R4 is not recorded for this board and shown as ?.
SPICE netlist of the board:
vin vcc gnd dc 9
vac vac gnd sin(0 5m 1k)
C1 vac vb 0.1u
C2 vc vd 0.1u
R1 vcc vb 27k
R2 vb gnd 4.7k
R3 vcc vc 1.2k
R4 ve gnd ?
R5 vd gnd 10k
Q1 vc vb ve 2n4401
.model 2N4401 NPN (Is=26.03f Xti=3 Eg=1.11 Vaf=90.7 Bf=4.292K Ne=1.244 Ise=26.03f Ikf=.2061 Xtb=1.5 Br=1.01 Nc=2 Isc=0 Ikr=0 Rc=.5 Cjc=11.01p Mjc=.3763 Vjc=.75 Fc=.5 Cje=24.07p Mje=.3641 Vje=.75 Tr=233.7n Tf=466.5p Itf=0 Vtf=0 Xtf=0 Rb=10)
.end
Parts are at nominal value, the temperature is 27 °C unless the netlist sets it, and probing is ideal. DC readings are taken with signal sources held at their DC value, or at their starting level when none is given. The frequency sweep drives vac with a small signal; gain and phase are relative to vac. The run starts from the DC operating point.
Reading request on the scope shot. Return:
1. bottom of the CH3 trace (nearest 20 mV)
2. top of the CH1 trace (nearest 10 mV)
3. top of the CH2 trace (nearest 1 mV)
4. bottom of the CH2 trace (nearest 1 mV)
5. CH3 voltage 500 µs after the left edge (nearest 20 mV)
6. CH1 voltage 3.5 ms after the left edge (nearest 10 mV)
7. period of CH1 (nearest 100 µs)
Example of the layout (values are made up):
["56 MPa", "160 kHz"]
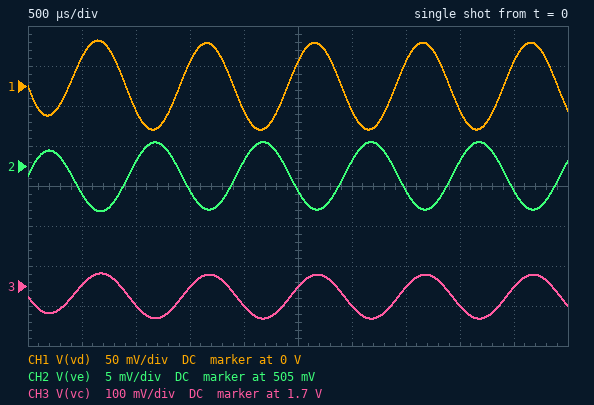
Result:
["1.62 V", "60 mV", "508 mV", "499 mV", "1.70 V", "30 mV", "1.0 ms"]
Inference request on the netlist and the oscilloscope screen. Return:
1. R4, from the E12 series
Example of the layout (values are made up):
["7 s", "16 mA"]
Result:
["82 Ω"]
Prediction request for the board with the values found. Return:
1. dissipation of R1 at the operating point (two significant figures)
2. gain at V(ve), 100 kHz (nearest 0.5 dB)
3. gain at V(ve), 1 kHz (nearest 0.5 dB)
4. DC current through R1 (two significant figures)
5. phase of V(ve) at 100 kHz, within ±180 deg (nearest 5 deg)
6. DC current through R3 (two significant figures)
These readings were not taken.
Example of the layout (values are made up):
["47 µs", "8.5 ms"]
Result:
["2.3 mW", "-0.5 dB", "-1.5 dB", "290 µA", "0 deg", "6.1 mA"]
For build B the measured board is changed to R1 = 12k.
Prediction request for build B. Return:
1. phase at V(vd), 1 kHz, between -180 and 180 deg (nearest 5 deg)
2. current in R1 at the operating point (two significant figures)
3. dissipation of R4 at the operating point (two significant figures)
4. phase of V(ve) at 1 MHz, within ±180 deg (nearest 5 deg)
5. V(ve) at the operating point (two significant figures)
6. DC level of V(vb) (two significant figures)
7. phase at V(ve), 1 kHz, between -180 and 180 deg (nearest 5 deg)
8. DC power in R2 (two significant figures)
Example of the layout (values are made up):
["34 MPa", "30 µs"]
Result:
["95 deg", "640 µA", "4.4 mW", "0 deg", "600 mV", "1.3 V", "85 deg", "350 µW"]
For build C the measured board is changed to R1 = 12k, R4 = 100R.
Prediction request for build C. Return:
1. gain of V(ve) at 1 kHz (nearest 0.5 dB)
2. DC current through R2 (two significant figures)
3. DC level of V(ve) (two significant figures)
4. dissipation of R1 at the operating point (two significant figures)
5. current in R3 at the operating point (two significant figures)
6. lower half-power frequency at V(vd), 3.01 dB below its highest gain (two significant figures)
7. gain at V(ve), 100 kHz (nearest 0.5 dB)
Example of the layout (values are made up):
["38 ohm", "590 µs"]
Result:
["-24.5 dB", "300 µA", "720 mV", "4.8 mW", "6.8 mA", "720 kHz", "-1.5 dB"]
